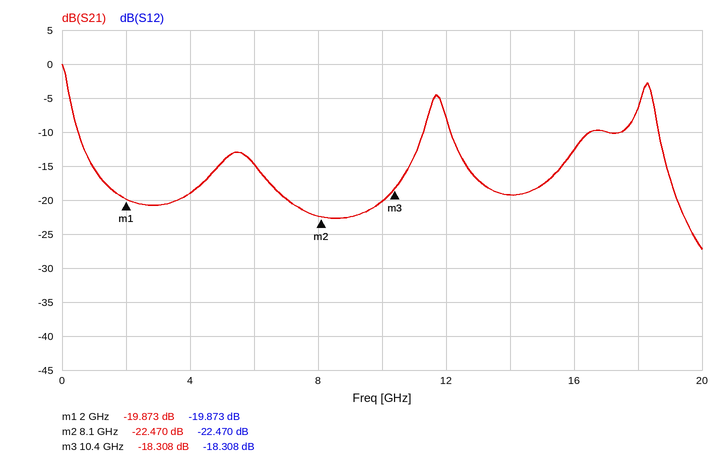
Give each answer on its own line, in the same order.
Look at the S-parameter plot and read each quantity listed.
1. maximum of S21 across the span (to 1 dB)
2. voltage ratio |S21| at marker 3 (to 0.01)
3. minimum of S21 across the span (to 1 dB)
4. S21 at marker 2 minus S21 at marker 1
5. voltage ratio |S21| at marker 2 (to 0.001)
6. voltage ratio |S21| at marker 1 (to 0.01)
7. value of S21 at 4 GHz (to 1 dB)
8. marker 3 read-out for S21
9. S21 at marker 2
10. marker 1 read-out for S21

0 dB
0.12
-27 dB
-2.597 dB
0.075
0.10
-19 dB
-18.308 dB
-22.470 dB
-19.873 dB
